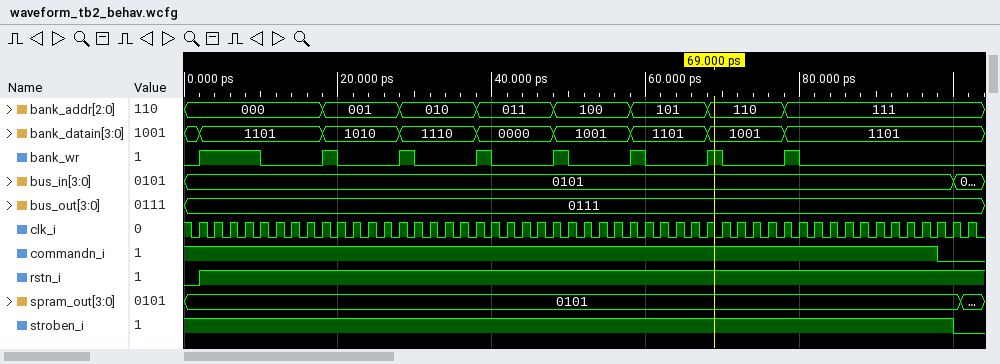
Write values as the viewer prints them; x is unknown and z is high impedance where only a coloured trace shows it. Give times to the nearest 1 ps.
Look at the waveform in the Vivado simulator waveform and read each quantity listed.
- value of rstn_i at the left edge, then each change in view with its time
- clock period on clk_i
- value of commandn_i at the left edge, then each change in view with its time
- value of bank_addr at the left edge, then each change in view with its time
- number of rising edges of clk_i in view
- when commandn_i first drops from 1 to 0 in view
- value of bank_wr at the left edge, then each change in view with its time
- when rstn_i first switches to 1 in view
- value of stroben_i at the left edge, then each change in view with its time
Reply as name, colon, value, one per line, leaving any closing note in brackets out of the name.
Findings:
value of rstn_i at the left edge, then each change in view with its time: 0, 1 at 2 ps
clock period on clk_i: 2 ps
value of commandn_i at the left edge, then each change in view with its time: 1, 0 at 98 ps
value of bank_addr at the left edge, then each change in view with its time: 000, 001 at 18 ps, 010 at 28 ps, 011 at 38 ps, 100 at 48 ps, 101 at 58 ps, 110 at 68 ps, 111 at 78 ps
number of rising edges of clk_i in view: 51
when commandn_i first drops from 1 to 0 in view: 98 ps
value of bank_wr at the left edge, then each change in view with its time: 0, 1 at 2 ps, 0 at 10 ps, 1 at 18 ps, 0 at 20 ps, 1 at 28 ps, 0 at 30 ps, 1 at 38 ps, 0 at 40 ps, 1 at 48 ps, 0 at 50 ps, 1 at 58 ps, 0 at 60 ps, 1 at 68 ps, 0 at 70 ps, 1 at 78 ps, 0 at 80 ps
when rstn_i first switches to 1 in view: 2 ps
value of stroben_i at the left edge, then each change in view with its time: 1, 0 at 100 ps
